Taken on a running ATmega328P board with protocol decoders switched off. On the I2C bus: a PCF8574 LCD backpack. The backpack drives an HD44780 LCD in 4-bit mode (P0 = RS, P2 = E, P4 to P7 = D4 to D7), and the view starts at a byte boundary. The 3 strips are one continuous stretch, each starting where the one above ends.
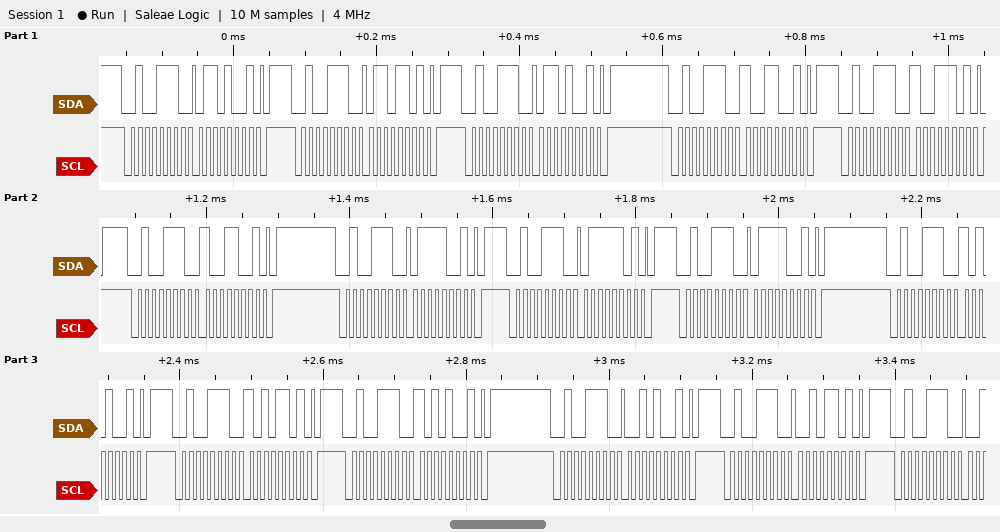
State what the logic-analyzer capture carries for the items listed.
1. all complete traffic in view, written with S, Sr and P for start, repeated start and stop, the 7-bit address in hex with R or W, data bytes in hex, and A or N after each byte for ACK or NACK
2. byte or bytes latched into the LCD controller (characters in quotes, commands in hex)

S 27W A 69 A P S 27W A 6D A P S 27W A 69 A P S 27W A 99 A P S 27W A 9D A P S 27W A 99 A P S 27W A 79 A P S 27W A 7D A P S 27W A 79 A P S 27W A A9 A P S 27W A AD A P S 27W A A9 A P S 27W A 29 A P S 27W A 2D A P S 27W A
'i' 'z'
